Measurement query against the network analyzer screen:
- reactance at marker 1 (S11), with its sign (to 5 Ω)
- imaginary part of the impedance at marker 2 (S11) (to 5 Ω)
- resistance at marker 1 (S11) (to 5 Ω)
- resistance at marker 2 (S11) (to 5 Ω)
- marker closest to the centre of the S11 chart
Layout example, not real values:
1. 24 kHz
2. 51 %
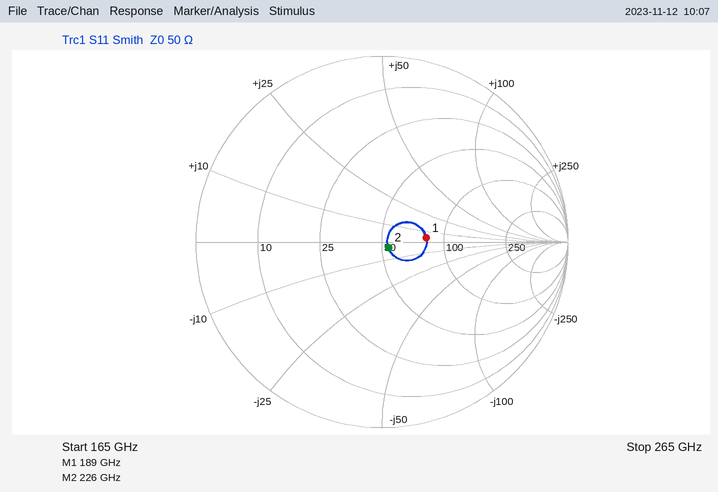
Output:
1. +5 Ω
2. -5 Ω
3. 80 Ω
4. 55 Ω
5. marker 2
